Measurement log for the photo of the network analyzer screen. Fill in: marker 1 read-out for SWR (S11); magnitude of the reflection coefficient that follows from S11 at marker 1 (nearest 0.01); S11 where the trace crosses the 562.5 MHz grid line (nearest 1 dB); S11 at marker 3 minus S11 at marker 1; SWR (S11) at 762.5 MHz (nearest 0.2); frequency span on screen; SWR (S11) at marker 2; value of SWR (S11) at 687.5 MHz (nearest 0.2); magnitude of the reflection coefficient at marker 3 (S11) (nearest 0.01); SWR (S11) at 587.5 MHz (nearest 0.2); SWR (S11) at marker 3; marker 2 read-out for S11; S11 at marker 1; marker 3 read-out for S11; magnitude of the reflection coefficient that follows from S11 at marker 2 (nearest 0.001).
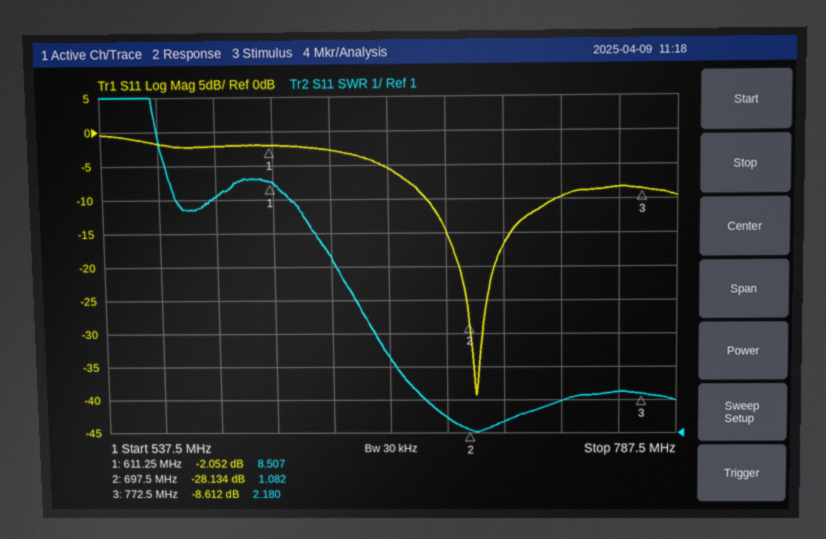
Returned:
8.507
0.79
-2 dB
-6.560 dB
2.2
250 MHz
1.082
1.4
0.37
8.0
2.180
-28.134 dB
-2.052 dB
-8.612 dB
0.039
